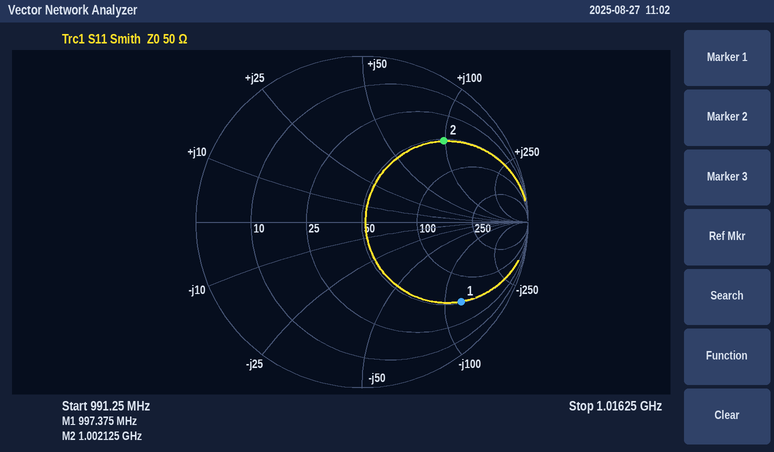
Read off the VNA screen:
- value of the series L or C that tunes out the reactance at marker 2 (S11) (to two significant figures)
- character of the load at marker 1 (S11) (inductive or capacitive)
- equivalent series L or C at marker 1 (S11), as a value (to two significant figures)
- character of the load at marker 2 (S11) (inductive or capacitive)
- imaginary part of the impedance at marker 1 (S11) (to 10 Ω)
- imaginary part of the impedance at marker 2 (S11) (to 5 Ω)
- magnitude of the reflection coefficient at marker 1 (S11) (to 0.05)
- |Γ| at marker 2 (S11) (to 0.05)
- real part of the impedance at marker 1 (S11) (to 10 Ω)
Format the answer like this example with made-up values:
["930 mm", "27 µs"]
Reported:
["1.6 pF", "capacitive", "1.3 pF", "inductive", "-120 Ω", "+100 Ω", "0.75", "0.70", "50 Ω"]
